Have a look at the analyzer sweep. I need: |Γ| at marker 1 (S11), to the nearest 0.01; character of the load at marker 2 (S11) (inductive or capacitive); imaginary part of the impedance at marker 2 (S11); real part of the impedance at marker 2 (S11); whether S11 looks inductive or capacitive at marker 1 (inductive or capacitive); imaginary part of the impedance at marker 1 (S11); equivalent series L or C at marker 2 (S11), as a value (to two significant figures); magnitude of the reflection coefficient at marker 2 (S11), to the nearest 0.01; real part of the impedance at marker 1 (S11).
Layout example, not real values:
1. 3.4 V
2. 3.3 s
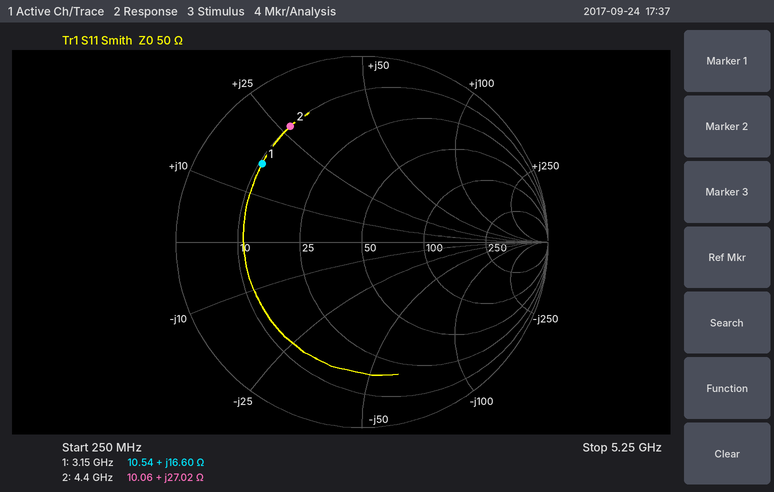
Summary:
1. 0.68
2. inductive
3. +27.02 Ω
4. 10.06 Ω
5. inductive
6. +16.60 Ω
7. 980 pH
8. 0.73
9. 10.54 Ω
